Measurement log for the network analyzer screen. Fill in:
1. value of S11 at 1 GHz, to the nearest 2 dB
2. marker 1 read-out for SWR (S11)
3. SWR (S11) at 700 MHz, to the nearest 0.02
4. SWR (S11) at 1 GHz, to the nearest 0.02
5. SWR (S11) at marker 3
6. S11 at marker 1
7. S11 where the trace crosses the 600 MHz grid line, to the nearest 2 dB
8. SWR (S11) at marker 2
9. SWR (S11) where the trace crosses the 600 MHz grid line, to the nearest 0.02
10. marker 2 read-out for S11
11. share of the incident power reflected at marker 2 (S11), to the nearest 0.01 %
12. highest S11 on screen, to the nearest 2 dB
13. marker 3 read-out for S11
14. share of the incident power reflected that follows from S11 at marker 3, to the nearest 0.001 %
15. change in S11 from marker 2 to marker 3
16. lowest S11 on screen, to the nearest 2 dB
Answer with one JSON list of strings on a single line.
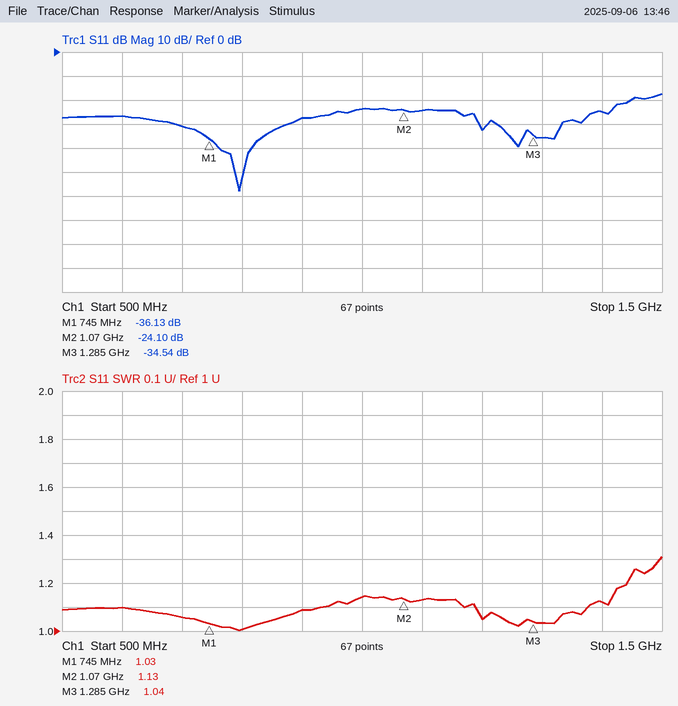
["-24 dB", "1.03", "1.06", "1.14", "1.04", "-36.13 dB", "-26 dB", "1.13", "1.10", "-24.10 dB", "0.39 %", "-18 dB", "-34.54 dB", "0.035 %", "-10.44 dB", "-58 dB"]
